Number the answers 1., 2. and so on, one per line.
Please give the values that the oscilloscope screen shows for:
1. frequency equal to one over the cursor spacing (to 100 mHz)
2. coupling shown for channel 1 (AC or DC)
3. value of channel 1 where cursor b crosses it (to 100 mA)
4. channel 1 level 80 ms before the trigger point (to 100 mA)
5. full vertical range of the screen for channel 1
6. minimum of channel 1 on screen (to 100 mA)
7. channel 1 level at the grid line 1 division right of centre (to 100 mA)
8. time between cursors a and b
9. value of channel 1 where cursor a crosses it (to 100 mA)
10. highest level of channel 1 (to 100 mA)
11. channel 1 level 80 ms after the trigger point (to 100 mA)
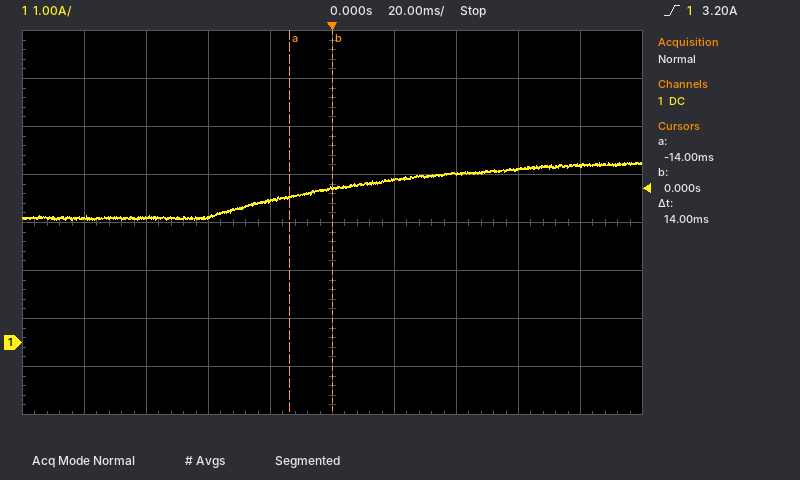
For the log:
1. 71.4 Hz
2. DC
3. 3.2 A
4. 2.6 A
5. 8 A
6. 2.5 A
7. 3.4 A
8. 14 ms
9. 3.0 A
10. 3.8 A
11. 3.7 A
